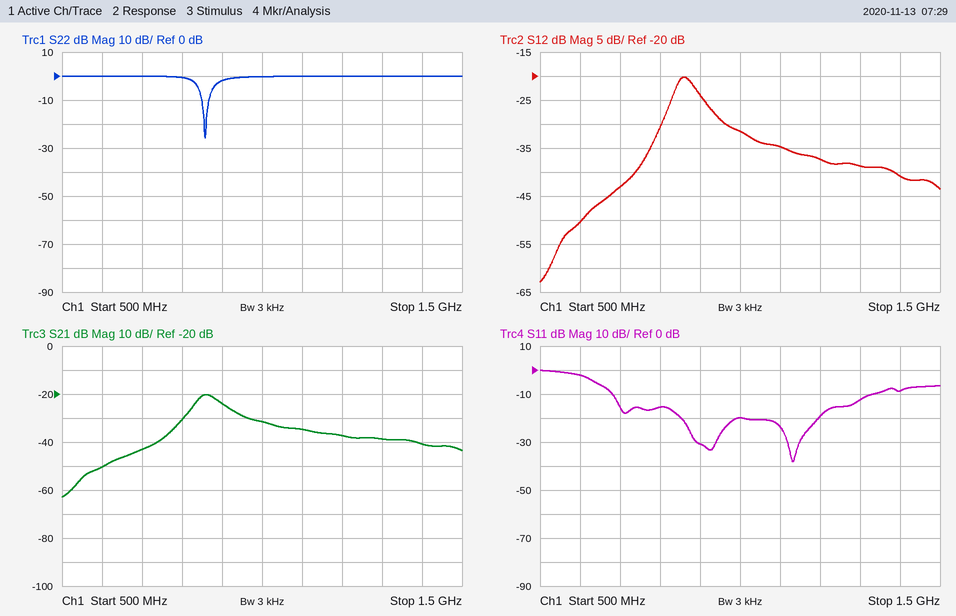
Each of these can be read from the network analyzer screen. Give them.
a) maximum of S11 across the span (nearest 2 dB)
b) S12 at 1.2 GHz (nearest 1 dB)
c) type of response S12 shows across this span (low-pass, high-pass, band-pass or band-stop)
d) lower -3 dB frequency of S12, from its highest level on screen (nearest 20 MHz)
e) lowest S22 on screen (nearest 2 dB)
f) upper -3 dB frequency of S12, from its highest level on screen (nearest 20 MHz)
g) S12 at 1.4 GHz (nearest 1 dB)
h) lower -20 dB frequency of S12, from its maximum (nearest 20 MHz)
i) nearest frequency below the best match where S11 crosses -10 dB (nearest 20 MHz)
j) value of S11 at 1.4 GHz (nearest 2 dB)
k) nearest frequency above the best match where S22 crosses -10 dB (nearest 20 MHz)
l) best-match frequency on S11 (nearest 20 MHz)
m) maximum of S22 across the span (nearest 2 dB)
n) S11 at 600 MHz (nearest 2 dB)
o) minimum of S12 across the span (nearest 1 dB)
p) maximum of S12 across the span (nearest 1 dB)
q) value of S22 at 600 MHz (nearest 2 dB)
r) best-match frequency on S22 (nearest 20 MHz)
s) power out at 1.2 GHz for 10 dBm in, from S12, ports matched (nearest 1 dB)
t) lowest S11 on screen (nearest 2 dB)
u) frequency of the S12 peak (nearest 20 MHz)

0 dB
-37 dB
band-pass
840 MHz
-26 dB
900 MHz
-41 dB
740 MHz
680 MHz
-8 dB
860 MHz
1.14 GHz
0 dB
-2 dB
-63 dB
-20 dB
0 dB
860 MHz
-27 dBm
-38 dB
860 MHz
